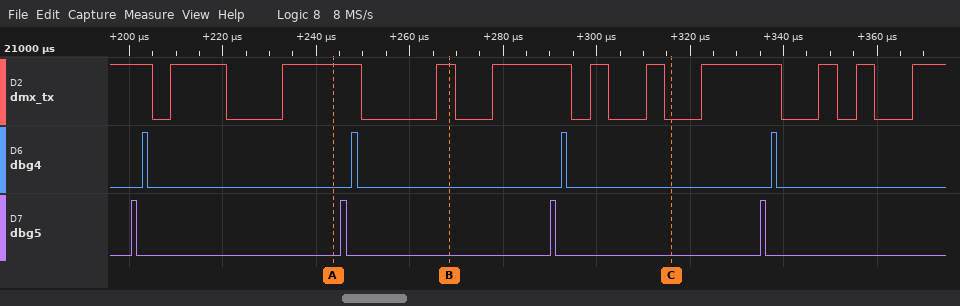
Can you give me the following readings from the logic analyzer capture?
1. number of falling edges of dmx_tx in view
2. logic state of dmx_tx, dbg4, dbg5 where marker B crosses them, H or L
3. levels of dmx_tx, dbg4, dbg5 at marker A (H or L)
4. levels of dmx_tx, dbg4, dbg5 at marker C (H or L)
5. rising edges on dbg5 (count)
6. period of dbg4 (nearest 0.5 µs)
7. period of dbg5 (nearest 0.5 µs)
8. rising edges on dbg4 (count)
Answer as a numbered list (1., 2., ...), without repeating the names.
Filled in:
1. 10
2. dmx_tx=H, dbg4=L, dbg5=L
3. dmx_tx=H, dbg4=L, dbg5=L
4. dmx_tx=L, dbg4=L, dbg5=L
5. 4
6. 45 µs
7. 45 µs
8. 4
